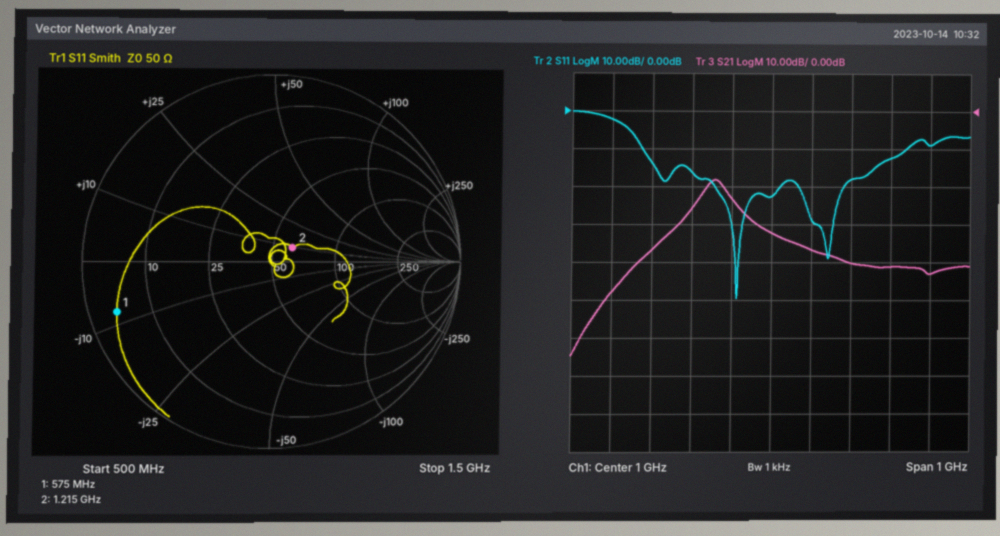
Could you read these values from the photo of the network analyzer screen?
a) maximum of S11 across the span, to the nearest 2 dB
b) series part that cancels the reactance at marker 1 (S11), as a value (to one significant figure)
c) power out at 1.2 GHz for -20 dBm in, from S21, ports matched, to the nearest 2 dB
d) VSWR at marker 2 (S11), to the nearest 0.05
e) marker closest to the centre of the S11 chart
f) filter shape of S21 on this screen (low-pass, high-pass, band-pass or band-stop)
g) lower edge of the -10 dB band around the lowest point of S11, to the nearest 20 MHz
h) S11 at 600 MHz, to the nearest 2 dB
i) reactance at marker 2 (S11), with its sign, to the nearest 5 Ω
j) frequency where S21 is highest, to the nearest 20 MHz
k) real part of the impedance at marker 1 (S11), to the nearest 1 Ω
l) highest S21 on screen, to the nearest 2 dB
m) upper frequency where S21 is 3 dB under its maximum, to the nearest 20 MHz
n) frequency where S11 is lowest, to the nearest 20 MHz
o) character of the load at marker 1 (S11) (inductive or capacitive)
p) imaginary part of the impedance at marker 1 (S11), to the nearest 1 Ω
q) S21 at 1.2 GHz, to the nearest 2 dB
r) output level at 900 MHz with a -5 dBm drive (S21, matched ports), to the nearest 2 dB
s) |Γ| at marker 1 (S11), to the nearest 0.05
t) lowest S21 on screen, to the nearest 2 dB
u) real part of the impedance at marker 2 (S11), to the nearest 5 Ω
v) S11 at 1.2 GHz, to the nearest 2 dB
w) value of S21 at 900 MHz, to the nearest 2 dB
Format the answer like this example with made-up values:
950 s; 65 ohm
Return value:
0 dB; 2 nH; -60 dBm; 1.30; marker 2; band-pass; 680 MHz; -2 dB; +10 Ω; 860 MHz; 4 Ω; -18 dB; 880 MHz; 920 MHz; capacitive; -8 Ω; -40 dB; -28 dBm; 0.85; -64 dB; 60 Ω; -18 dB; -24 dB
